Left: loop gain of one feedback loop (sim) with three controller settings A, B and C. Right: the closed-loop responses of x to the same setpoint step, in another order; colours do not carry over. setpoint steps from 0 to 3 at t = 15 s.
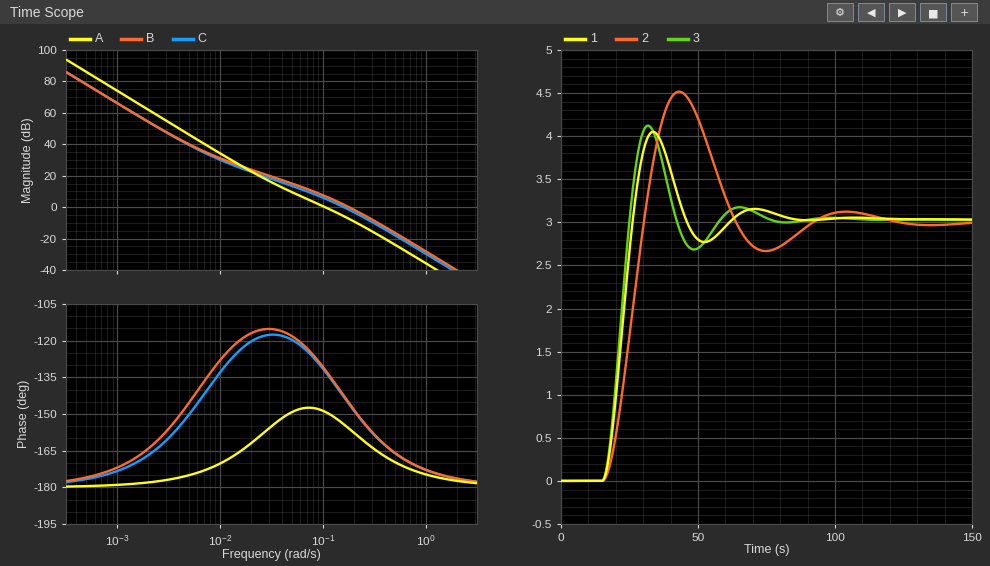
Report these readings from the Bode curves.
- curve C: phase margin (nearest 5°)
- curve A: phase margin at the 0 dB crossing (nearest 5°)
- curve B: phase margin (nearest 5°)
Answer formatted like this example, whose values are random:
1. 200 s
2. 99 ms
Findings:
1. 35°
2. 30°
3. 35°
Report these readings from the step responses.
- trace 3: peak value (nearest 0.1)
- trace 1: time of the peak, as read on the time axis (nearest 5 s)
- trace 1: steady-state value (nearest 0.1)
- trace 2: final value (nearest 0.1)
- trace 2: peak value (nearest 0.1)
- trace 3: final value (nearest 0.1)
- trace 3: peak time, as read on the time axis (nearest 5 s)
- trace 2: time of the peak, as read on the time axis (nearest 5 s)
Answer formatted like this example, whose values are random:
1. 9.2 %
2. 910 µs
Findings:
1. 4.1
2. 35 s
3. 3.0
4. 3.0
5. 4.5
6. 3.0
7. 30 s
8. 45 s
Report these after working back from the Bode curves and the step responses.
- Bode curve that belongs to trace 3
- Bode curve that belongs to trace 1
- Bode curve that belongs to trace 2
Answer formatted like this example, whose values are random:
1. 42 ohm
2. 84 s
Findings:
1. B
2. C
3. A
